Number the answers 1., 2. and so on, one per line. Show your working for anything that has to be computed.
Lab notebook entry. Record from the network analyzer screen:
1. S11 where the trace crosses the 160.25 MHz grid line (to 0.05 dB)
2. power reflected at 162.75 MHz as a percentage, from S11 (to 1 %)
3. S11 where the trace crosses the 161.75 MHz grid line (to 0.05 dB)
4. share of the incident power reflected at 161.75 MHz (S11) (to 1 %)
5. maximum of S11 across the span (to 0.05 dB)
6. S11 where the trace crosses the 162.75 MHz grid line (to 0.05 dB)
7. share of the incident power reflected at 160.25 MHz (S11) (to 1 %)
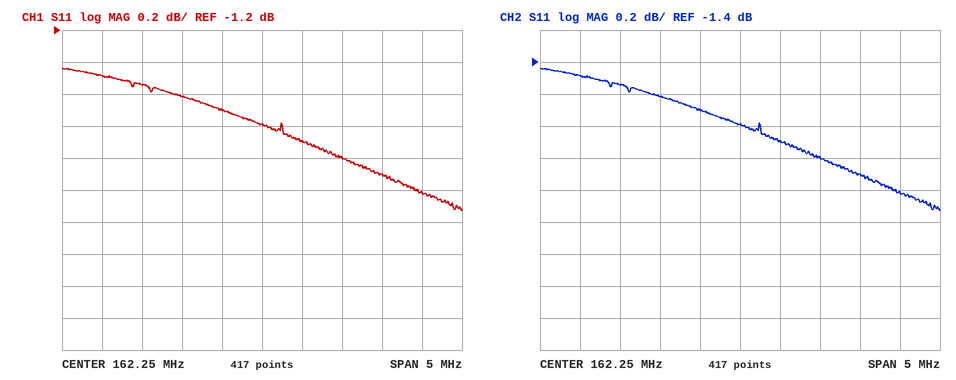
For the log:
1. -1.50 dB
2. 10^(-1.9/10) ≈ 65 %
3. -1.70 dB
4. 10^(-1.7/10) ≈ 68 %
5. -1.45 dB
6. -1.90 dB
7. 10^(-1.5/10) ≈ 71 %
